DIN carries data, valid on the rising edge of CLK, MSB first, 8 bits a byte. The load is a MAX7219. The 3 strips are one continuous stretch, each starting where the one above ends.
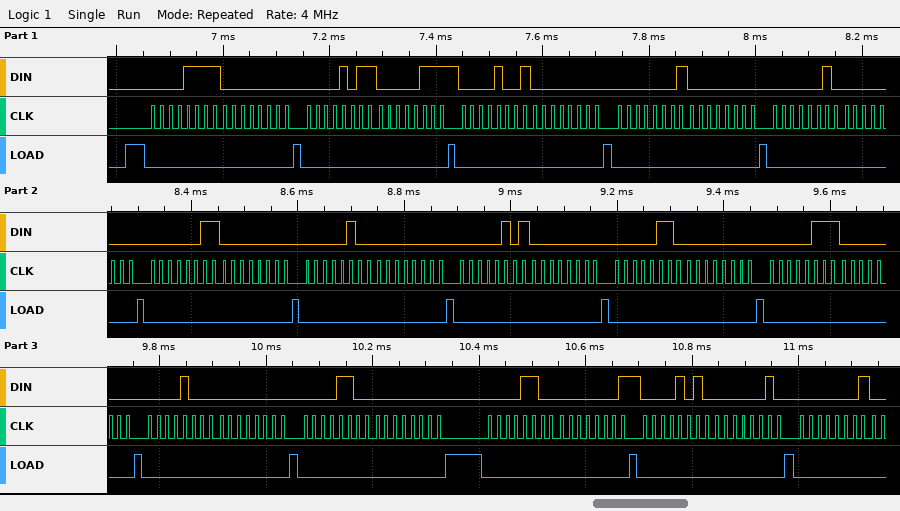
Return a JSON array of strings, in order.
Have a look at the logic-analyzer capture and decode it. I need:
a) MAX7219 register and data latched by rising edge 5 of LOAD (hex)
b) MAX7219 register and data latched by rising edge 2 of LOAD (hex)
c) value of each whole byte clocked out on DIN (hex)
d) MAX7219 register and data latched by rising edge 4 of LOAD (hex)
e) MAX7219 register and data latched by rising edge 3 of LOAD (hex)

["register 0x1, data 0x00", "register 0xF, data 0x00", "0F 00 0B 07 09 00 01 00 02 00 03 00 04 00 05 00 06 00 07 00 08 00 0C 00 0C 01 0A 02 01", "register 0x9, data 0x00", "register 0xB, data 0x07"]
